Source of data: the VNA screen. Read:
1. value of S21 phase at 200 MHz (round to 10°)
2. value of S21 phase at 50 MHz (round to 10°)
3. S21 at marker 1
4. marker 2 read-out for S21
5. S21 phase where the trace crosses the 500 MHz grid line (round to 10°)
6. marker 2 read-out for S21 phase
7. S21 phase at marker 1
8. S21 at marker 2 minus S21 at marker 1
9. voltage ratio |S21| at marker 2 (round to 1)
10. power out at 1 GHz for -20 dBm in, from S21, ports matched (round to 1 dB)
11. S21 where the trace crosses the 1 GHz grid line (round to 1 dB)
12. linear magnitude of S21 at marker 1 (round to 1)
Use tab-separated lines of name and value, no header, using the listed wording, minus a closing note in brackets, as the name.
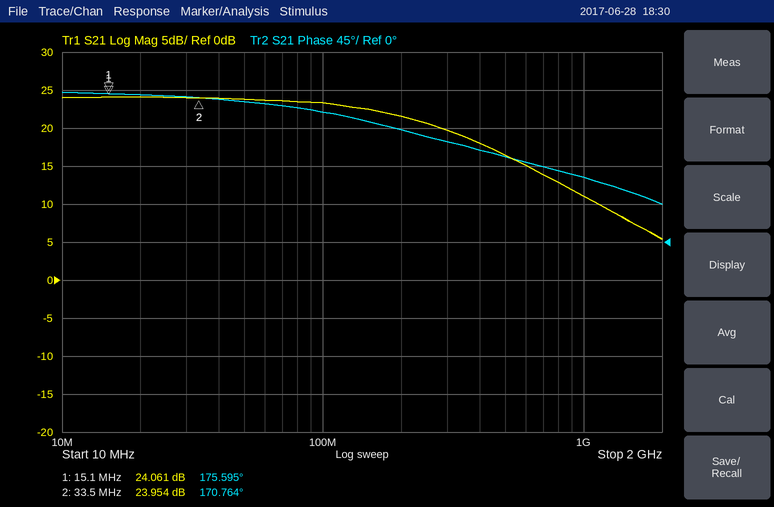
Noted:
value of S21 phase at 200 MHz	130°
value of S21 phase at 50 MHz	170°
S21 at marker 1	24.061 dB
marker 2 read-out for S21	23.954 dB
S21 phase where the trace crosses the 500 MHz grid line	100°
marker 2 read-out for S21 phase	170.764°
S21 phase at marker 1	175.595°
S21 at marker 2 minus S21 at marker 1	-0.107 dB
voltage ratio |S21| at marker 2	16
power out at 1 GHz for -20 dBm in, from S21, ports matched	-9 dBm
S21 where the trace crosses the 1 GHz grid line	11 dB
linear magnitude of S21 at marker 1	16
